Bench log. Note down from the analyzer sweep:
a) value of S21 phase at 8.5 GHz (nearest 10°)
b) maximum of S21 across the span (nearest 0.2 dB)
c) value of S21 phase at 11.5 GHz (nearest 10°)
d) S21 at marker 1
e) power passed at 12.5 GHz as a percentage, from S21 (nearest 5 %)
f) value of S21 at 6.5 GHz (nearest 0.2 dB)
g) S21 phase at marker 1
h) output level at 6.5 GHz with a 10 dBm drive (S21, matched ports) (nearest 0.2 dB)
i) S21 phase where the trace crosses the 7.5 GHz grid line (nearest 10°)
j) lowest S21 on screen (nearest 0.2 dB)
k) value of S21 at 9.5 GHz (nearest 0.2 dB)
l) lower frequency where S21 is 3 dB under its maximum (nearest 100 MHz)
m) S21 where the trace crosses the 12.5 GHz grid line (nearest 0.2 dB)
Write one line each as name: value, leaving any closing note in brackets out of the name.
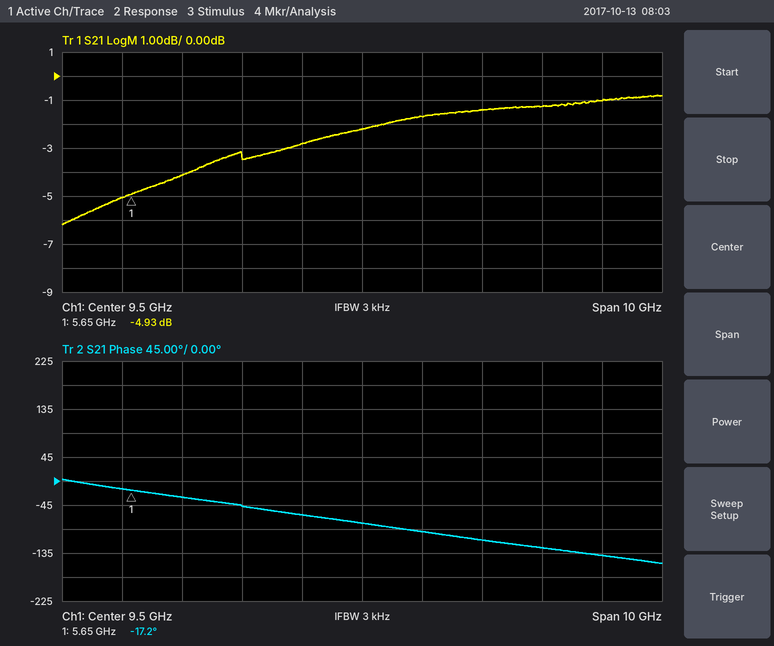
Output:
value of S21 phase at 8.5 GHz: -60°
maximum of S21 across the span: -0.8 dB
value of S21 phase at 11.5 GHz: -110°
S21 at marker 1: -4.93 dB
power passed at 12.5 GHz as a percentage, from S21: 75 %
value of S21 at 6.5 GHz: -4.2 dB
S21 phase at marker 1: -17.2°
output level at 6.5 GHz with a 10 dBm drive (S21, matched ports): 5.8 dBm
S21 phase where the trace crosses the 7.5 GHz grid line: -50°
lowest S21 on screen: -6.2 dB
value of S21 at 9.5 GHz: -2.2 dB
lower frequency where S21 is 3 dB under its maximum: 6.8 GHz
S21 where the trace crosses the 12.5 GHz grid line: -1.2 dB
